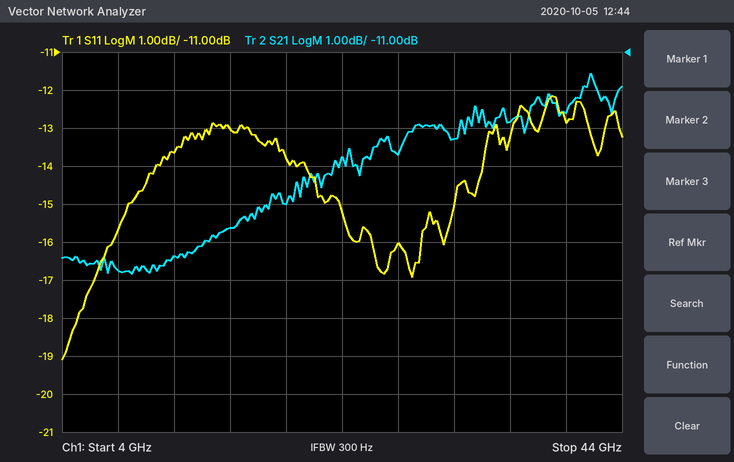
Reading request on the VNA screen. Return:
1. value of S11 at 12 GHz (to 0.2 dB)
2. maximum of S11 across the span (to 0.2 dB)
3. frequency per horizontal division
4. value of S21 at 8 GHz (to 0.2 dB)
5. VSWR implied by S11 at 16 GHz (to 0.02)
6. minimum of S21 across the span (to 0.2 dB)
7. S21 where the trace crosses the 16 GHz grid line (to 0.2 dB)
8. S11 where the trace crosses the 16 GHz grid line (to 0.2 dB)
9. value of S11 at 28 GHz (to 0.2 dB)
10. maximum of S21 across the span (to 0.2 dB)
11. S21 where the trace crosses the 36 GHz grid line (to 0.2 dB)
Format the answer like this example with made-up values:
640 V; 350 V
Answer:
-13.6 dB; -12.2 dB; 4 GHz; -16.8 dB; 1.58; -16.8 dB; -15.6 dB; -13.0 dB; -16.0 dB; -11.6 dB; -12.8 dB
